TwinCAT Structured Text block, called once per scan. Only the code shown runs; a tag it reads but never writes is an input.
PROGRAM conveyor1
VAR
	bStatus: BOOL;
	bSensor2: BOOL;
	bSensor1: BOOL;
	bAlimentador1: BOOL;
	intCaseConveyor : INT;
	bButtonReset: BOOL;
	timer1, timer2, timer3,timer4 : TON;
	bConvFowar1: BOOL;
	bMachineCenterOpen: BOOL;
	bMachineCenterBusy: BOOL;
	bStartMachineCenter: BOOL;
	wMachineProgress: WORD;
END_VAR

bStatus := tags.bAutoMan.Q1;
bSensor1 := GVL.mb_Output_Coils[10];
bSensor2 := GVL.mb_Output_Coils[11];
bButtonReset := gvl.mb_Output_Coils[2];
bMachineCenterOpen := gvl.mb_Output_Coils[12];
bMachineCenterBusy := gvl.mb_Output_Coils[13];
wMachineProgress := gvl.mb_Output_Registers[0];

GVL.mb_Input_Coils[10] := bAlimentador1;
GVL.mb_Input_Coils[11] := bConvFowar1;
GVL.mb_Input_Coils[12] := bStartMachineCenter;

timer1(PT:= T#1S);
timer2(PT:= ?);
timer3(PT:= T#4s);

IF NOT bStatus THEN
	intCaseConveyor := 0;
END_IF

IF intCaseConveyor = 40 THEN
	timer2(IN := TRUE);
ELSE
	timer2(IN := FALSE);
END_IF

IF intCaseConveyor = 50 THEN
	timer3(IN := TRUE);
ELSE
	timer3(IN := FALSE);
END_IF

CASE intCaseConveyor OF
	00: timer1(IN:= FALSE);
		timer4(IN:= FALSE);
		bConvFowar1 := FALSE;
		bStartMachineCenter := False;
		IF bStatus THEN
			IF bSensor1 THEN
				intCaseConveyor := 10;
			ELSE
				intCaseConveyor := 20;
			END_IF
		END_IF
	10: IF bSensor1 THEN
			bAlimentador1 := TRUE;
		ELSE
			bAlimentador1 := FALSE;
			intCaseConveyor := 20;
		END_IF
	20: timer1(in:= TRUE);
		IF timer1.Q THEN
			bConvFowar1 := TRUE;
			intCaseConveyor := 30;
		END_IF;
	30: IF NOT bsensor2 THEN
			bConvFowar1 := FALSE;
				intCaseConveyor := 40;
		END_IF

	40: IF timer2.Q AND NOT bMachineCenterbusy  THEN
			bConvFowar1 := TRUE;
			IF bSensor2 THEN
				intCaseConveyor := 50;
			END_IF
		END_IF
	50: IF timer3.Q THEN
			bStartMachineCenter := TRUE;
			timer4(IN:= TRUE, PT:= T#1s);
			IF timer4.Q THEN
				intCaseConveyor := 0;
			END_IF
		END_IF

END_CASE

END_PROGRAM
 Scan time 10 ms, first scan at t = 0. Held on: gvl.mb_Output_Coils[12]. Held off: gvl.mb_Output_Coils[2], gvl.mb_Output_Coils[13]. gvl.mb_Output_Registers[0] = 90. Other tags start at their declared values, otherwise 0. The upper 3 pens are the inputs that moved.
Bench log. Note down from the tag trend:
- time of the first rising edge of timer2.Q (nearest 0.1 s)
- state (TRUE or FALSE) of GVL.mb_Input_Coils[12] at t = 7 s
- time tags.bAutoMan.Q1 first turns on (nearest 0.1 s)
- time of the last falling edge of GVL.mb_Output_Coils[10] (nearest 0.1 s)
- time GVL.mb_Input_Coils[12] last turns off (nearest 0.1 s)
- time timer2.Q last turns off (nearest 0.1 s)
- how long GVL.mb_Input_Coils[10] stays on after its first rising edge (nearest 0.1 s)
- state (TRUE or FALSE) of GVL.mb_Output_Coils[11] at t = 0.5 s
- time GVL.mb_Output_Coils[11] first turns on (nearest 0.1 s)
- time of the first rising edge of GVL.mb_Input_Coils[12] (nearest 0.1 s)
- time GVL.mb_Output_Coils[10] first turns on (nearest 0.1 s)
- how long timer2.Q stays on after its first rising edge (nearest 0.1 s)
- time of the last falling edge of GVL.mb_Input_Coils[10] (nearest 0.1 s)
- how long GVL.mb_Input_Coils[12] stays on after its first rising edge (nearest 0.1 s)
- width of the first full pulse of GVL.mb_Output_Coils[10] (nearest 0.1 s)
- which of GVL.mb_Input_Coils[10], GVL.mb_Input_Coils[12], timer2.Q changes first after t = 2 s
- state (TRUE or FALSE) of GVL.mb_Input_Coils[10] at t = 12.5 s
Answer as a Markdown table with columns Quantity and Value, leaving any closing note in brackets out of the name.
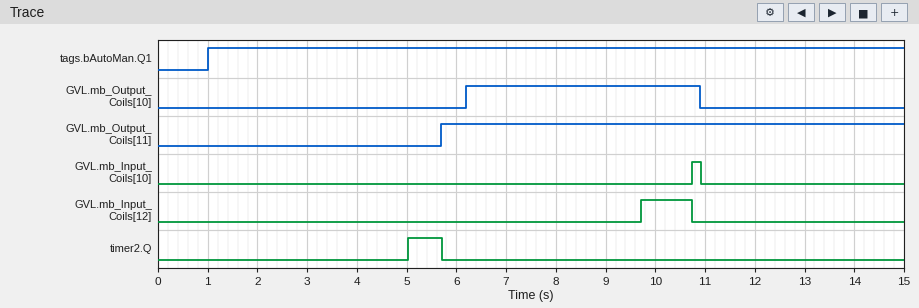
| Quantity | Value |
|---|---|
| time of the first rising edge of timer2.Q | 5.0 s |
| state (TRUE or FALSE) of GVL.mb_Input_Coils[12] at t = 7 s | FALSE |
| time tags.bAutoMan.Q1 first turns on | 1.0 s |
| time of the last falling edge of GVL.mb_Output_Coils[10] | 10.9 s |
| time GVL.mb_Input_Coils[12] last turns off | 10.7 s |
| time timer2.Q last turns off | 5.7 s |
| how long GVL.mb_Input_Coils[10] stays on after its first rising edge | 0.2 s |
| state (TRUE or FALSE) of GVL.mb_Output_Coils[11] at t = 0.5 s | FALSE |
| time GVL.mb_Output_Coils[11] first turns on | 5.7 s |
| time of the first rising edge of GVL.mb_Input_Coils[12] | 9.7 s |
| time GVL.mb_Output_Coils[10] first turns on | 6.2 s |
| how long timer2.Q stays on after its first rising edge | 0.7 s |
| time of the last falling edge of GVL.mb_Input_Coils[10] | 10.9 s |
| how long GVL.mb_Input_Coils[12] stays on after its first rising edge | 1.0 s |
| width of the first full pulse of GVL.mb_Output_Coils[10] | 4.7 s |
| which of GVL.mb_Input_Coils[10], GVL.mb_Input_Coils[12], timer2.Q changes first after t = 2 s | timer2.Q |
| state (TRUE or FALSE) of GVL.mb_Input_Coils[10] at t = 12.5 s | FALSE |
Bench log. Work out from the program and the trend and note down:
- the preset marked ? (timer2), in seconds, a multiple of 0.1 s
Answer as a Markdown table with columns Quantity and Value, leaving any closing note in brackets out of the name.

| Quantity | Value |
|---|---|
| the preset marked ? (timer2), in seconds, a multiple of 0.1 s | 3.0 s |
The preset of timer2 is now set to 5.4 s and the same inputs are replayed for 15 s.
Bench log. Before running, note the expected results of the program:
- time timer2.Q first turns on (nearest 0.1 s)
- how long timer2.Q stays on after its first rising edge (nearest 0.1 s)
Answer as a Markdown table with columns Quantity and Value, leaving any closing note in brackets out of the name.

| Quantity | Value |
|---|---|
| time timer2.Q first turns on | 7.4 s |
| how long timer2.Q stays on after its first rising edge | 0.0 s |
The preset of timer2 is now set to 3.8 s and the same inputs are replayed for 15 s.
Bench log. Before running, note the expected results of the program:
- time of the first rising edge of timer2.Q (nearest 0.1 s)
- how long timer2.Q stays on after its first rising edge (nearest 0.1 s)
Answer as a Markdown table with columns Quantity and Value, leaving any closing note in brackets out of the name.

| Quantity | Value |
|---|---|
| time of the first rising edge of timer2.Q | 5.8 s |
| how long timer2.Q stays on after its first rising edge | 0.0 s |
